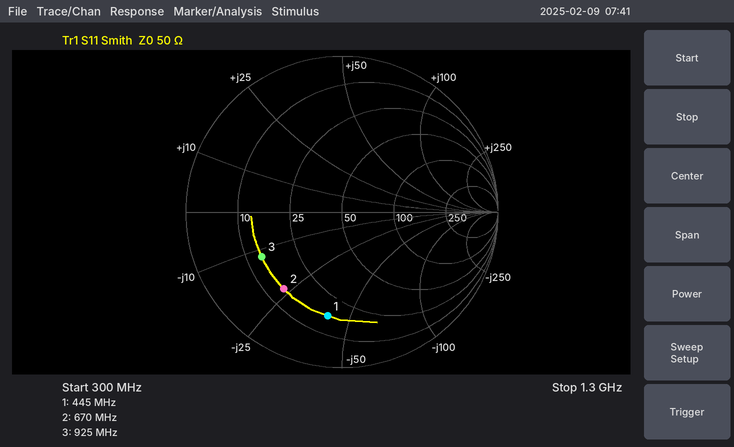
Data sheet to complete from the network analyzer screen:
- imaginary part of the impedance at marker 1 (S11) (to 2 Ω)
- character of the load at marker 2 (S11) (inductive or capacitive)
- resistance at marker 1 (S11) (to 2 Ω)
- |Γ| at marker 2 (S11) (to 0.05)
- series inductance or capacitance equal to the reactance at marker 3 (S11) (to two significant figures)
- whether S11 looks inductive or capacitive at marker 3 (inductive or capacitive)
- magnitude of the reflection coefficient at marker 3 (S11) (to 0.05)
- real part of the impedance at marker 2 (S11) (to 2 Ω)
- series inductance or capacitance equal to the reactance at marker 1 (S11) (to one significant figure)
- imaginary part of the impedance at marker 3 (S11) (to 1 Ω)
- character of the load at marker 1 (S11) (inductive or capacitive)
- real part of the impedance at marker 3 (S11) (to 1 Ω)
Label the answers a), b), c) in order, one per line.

a) -40 Ω
b) capacitive
c) 16 Ω
d) 0.60
e) 14 pF
f) capacitive
g) 0.60
h) 14 Ω
i) 9 pF
j) -12 Ω
k) capacitive
l) 14 Ω
